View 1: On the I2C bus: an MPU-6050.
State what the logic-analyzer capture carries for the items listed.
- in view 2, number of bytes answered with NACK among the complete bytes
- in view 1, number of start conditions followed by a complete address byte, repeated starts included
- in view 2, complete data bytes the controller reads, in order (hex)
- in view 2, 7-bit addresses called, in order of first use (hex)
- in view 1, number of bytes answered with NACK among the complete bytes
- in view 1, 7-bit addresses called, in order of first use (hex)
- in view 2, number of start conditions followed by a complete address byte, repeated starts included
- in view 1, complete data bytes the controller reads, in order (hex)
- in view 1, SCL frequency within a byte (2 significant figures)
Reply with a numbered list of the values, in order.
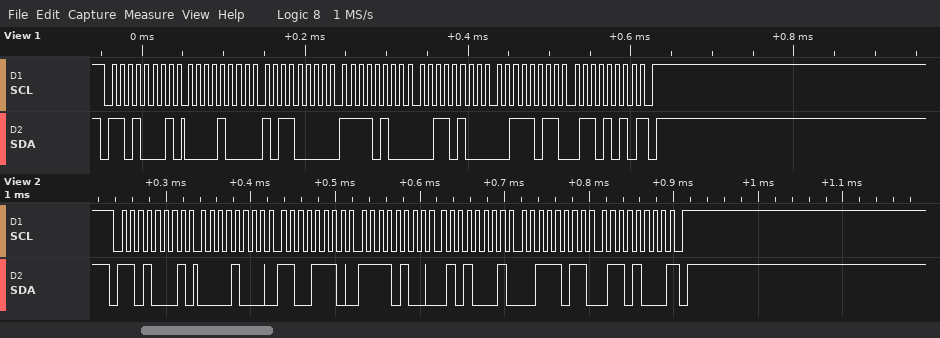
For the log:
1. 1
2. 1
3. 08 CE F4 51 3B 68
4. 0x68
5. 1
6. 0x68
7. 1
8. 08 B0 F4 34 3B 6A
9. 100 kHz
